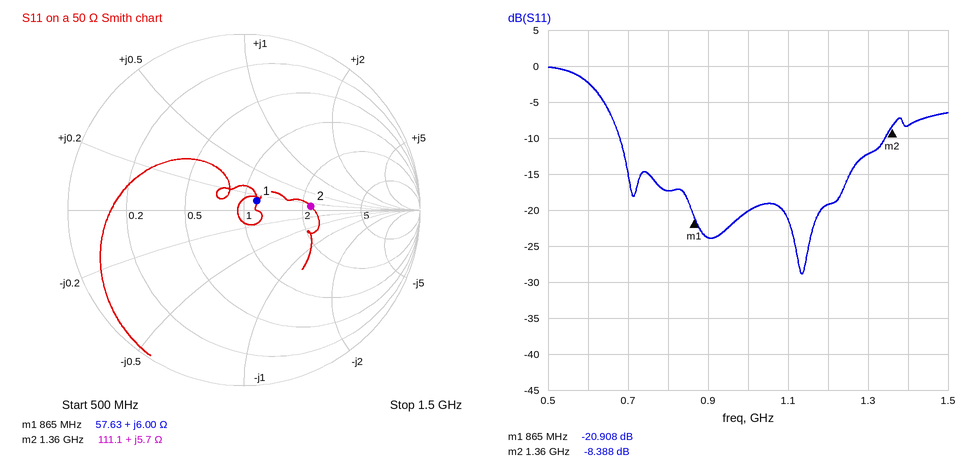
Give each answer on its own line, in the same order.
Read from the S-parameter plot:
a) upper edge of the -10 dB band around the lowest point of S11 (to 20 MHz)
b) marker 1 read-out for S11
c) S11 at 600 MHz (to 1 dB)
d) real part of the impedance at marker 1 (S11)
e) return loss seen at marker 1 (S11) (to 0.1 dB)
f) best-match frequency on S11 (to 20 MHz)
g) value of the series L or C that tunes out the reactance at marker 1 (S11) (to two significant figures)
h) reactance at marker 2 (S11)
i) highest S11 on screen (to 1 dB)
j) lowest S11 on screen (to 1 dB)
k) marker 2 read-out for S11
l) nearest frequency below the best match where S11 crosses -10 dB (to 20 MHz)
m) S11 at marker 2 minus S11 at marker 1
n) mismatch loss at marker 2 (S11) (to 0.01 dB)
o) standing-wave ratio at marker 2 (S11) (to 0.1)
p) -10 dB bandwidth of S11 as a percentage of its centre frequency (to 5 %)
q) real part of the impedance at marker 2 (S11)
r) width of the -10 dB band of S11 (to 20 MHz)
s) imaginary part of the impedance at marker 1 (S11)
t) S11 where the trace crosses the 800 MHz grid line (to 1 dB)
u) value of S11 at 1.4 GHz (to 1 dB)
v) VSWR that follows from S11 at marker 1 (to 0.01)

1.34 GHz
-20.908 dB
-2 dB
57.63 Ω
20.9 dB
1.14 GHz
31 pF
+5.7 Ω
0 dB
-29 dB
-8.388 dB
680 MHz
12.520 dB
0.68 dB
2.2
65 %
111.1 Ω
660 MHz
+6.00 Ω
-17 dB
-8 dB
1.20
